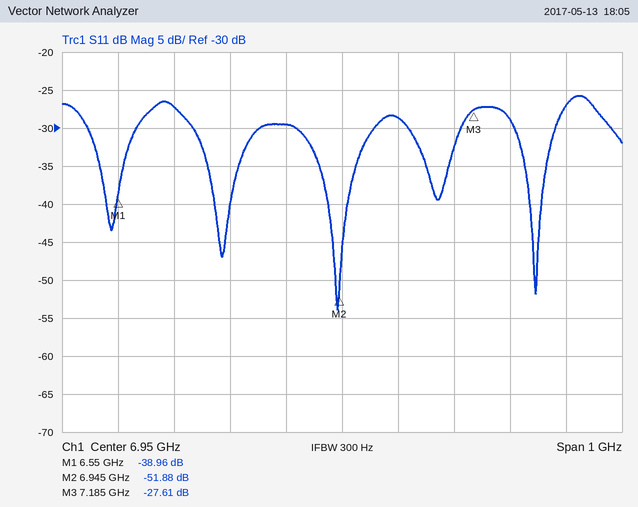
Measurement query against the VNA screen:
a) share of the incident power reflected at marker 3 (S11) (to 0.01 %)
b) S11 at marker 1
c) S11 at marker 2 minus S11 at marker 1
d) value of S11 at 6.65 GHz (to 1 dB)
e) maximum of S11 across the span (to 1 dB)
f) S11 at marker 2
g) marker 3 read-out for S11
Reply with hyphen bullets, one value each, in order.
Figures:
- 0.17 %
- -38.96 dB
- -12.92 dB
- -27 dB
- -26 dB
- -51.88 dB
- -27.61 dB
